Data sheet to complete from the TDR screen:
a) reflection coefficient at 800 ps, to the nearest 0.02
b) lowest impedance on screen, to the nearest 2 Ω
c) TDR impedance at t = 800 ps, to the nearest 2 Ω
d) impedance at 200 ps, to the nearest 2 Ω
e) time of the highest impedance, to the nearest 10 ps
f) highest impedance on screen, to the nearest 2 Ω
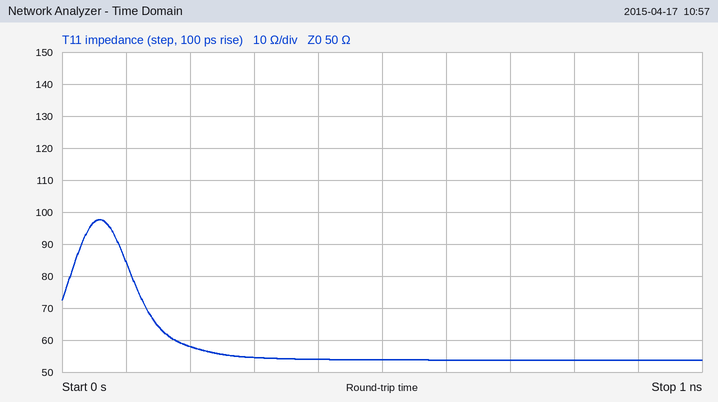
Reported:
+0.04
54 Ω
54 Ω
58 Ω
60 ps
98 Ω
